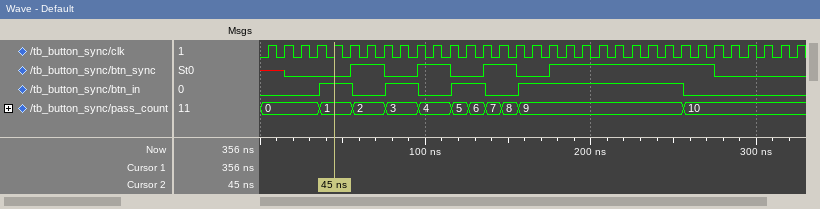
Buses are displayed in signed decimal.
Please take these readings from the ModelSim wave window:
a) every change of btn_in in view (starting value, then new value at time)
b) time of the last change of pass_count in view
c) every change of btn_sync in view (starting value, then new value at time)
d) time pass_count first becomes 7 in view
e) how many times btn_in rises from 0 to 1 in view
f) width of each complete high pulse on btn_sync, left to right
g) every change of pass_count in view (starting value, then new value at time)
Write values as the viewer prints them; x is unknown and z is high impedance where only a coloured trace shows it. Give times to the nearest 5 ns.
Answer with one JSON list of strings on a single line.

["0, 1 at 35 ns, 0 at 55 ns, 1 at 75 ns, 0 at 95 ns, 1 at 115 ns, 0 at 135 ns, 1 at 155 ns, 0 at 255 ns", "255 ns", "x, 0 at 15 ns, 1 at 55 ns, 0 at 75 ns, 1 at 95 ns, 0 at 115 ns, 1 at 135 ns, 0 at 155 ns, 1 at 175 ns, 0 at 275 ns", "135 ns", "4", "20 ns, 20 ns, 20 ns, 100 ns", "0, 1 at 35 ns, 2 at 55 ns, 3 at 75 ns, 4 at 95 ns, 5 at 115 ns, 6 at 125 ns, 7 at 135 ns, 8 at 145 ns, 9 at 155 ns, 10 at 255 ns"]
